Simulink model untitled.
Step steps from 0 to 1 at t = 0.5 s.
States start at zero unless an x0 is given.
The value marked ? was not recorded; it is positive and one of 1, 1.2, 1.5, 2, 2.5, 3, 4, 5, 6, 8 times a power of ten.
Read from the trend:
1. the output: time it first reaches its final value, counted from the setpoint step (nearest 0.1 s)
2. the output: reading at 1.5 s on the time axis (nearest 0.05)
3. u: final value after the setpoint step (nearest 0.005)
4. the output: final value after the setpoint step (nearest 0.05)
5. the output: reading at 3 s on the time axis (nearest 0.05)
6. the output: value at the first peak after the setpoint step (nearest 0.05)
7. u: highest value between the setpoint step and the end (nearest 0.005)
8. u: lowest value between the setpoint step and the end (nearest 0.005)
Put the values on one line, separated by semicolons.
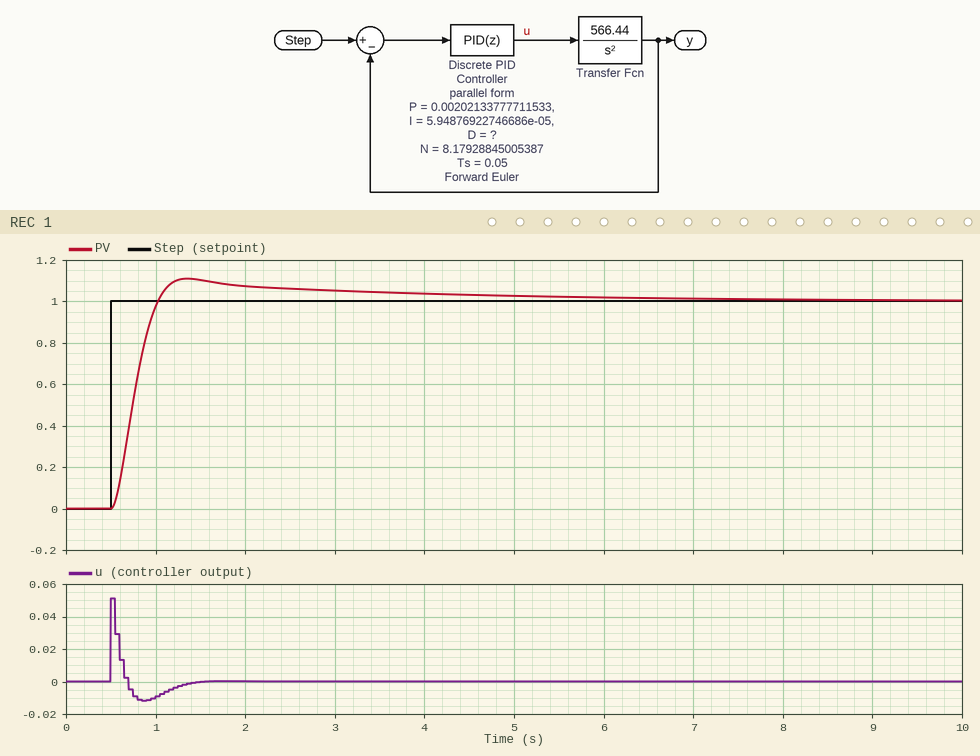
0.5 s; 1.10; 0.000; 1.00; 1.05; 1.10; 0.050; -0.010
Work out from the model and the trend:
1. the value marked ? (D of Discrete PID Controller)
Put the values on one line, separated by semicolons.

0.006
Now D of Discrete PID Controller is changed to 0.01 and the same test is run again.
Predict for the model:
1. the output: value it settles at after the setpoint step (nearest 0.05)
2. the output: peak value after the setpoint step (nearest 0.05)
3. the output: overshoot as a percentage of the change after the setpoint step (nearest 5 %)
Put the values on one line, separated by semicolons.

1.00; 1.15; 15 %
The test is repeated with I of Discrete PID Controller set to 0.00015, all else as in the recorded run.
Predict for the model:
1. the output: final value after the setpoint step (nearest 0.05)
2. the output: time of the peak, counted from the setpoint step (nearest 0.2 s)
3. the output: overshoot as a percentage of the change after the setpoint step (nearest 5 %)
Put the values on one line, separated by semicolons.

1.00; 0.8 s; 10 %
